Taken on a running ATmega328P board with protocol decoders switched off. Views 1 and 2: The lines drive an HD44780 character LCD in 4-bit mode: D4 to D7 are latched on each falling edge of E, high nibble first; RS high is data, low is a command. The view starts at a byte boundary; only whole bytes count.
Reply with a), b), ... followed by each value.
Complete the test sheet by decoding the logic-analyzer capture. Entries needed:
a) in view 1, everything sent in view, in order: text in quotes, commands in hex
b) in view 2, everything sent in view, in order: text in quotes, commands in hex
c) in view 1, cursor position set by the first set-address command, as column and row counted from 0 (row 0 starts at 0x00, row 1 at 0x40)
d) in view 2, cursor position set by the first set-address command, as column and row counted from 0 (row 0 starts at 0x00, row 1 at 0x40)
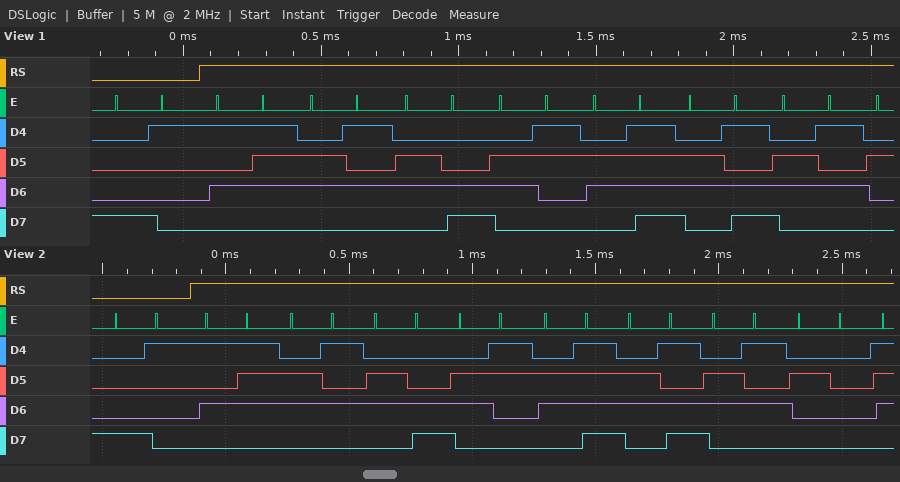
a) 0x81 "Welcome"
b) 0x81 "Welcome "
c) column 1, row 0
d) column 1, row 0
